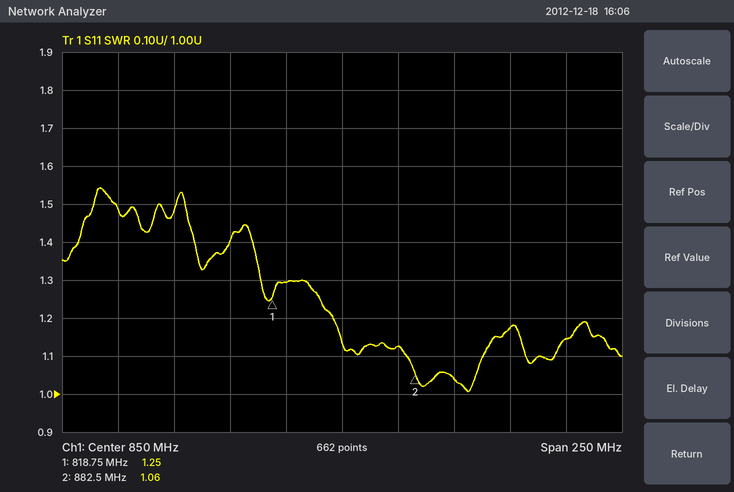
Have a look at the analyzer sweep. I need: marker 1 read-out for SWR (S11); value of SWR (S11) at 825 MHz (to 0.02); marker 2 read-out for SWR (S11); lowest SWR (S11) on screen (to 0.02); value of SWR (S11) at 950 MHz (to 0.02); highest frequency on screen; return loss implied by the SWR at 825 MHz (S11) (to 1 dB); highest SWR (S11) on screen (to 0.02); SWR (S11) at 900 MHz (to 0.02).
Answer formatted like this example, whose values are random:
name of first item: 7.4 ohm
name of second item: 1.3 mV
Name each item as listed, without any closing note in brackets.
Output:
marker 1 read-out for SWR: 1.25
value of SWR (S11) at 825 MHz: 1.30
marker 2 read-out for SWR: 1.06
lowest SWR (S11) on screen: 1.00
value of SWR (S11) at 950 MHz: 1.14
highest frequency on screen: 975 MHz
return loss implied by the SWR at 825 MHz (S11): 18 dB
highest SWR (S11) on screen: 1.54
SWR (S11) at 900 MHz: 1.04
